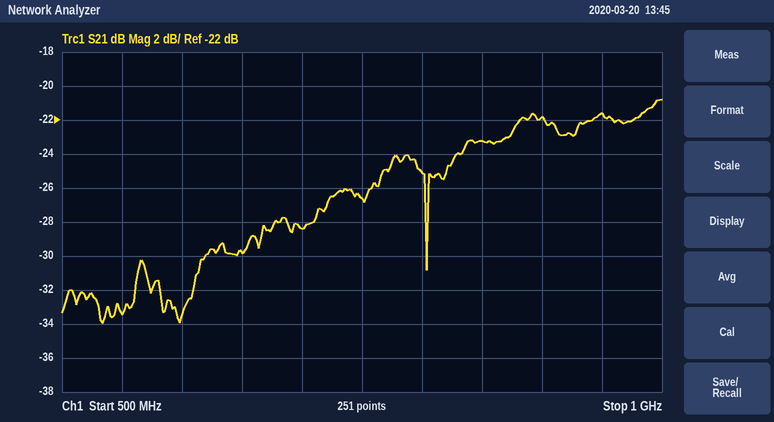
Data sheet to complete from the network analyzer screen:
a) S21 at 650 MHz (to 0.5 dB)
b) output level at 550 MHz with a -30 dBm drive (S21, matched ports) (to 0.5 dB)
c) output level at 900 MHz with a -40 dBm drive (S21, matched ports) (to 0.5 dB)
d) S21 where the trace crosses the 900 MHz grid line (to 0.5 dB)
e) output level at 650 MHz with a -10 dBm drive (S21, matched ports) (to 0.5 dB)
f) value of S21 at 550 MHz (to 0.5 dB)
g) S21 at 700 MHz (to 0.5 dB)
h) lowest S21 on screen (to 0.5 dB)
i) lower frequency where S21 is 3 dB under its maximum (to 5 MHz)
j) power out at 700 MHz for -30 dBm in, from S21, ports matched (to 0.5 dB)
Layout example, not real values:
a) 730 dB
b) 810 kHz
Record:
a) -30.0 dB
b) -63.5 dBm
c) -62.0 dBm
d) -22.0 dB
e) -40.0 dBm
f) -33.5 dB
g) -28.5 dB
h) -34.0 dB
i) 835 MHz
j) -58.5 dBm
